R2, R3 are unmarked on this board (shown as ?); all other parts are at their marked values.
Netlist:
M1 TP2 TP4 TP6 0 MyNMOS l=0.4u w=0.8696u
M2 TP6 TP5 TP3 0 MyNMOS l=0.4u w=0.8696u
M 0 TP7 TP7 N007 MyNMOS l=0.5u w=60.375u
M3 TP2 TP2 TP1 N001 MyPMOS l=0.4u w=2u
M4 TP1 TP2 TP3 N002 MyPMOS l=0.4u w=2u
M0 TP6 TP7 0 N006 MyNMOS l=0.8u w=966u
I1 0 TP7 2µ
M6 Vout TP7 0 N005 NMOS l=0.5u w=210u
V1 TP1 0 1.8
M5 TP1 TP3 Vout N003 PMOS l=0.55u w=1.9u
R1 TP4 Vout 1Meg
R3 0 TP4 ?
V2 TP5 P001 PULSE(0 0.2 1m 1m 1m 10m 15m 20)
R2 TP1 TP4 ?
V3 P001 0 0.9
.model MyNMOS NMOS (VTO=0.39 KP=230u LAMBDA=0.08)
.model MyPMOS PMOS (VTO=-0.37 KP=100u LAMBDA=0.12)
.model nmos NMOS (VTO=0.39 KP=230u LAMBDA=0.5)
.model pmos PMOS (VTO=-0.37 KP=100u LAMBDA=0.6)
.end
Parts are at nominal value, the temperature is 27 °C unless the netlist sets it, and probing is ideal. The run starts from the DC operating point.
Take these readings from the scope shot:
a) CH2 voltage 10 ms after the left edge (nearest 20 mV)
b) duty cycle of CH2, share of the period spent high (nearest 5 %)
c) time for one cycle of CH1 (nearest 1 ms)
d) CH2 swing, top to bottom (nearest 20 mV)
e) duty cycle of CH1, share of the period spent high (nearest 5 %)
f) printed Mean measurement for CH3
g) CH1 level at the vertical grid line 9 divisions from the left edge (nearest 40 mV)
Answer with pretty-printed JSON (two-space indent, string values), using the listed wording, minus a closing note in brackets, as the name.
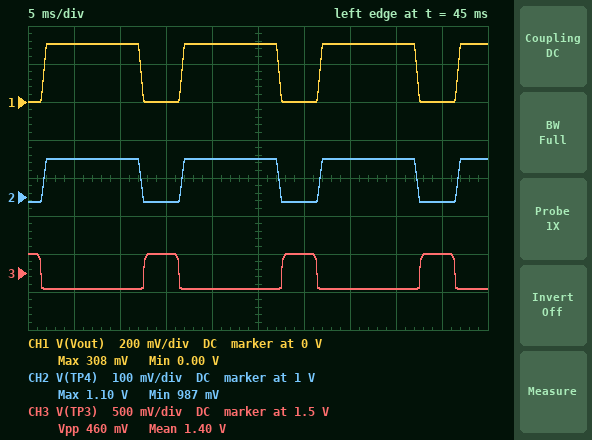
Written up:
{
  "CH2 voltage 10 ms after the left edge": "1.10 V",
  "duty cycle of CH2, share of the period spent high": "70 %",
  "time for one cycle of CH1": "15 ms",
  "CH2 swing, top to bottom": "120 mV",
  "duty cycle of CH1, share of the period spent high": "70 %",
  "printed Mean measurement for CH3": "1.40 V",
  "CH1 level at the vertical grid line 9 divisions from the left edge": "0 V"
}
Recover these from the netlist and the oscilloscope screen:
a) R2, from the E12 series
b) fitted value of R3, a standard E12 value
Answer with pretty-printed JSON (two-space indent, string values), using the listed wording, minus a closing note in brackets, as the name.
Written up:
{
  "R2, from the E12 series": "680 kΩ",
  "fitted value of R3, a standard E12 value": "4.7 MΩ"
}
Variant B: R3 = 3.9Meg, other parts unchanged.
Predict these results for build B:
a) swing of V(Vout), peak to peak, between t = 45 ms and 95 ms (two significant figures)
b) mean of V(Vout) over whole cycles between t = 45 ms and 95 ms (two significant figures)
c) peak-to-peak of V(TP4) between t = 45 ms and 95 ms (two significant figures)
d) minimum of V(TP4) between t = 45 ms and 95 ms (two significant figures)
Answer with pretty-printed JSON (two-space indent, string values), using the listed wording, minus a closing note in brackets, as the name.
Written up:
{
  "swing of V(Vout), peak to peak, between t = 45 ms and 95 ms": "350 mV",
  "mean of V(Vout) over whole cycles between t = 45 ms and 95 ms": "250 mV",
  "peak-to-peak of V(TP4) between t = 45 ms and 95 ms": "130 mV",
  "minimum of V(TP4) between t = 45 ms and 95 ms": "970 mV"
}
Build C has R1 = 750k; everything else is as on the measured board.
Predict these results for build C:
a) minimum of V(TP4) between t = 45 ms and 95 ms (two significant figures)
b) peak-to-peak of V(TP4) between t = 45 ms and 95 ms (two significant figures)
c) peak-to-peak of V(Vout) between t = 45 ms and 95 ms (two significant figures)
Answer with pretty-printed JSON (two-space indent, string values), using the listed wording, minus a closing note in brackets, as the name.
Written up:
{
  "minimum of V(TP4) between t = 45 ms and 95 ms": "900 mV",
  "peak-to-peak of V(TP4) between t = 45 ms and 95 ms": "200 mV",
  "peak-to-peak of V(Vout) between t = 45 ms and 95 ms": "450 mV"
}
